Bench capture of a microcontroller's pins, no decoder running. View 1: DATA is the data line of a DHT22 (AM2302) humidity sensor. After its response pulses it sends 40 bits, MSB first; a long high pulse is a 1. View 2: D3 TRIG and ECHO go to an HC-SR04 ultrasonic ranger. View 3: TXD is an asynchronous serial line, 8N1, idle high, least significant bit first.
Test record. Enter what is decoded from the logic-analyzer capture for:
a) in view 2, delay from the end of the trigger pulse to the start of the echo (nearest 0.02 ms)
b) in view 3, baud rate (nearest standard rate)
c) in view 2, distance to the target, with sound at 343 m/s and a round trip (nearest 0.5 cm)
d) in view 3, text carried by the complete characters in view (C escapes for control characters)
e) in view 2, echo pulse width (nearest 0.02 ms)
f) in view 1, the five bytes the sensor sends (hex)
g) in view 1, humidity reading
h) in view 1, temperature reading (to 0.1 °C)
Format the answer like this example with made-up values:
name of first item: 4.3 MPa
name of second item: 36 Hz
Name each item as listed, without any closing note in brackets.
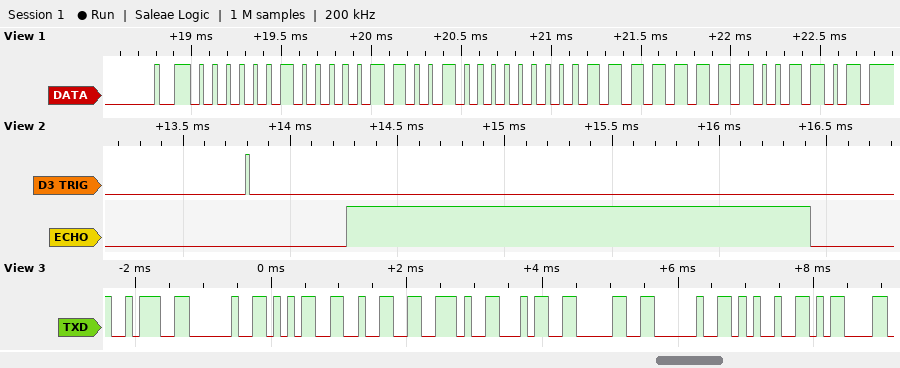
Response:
in view 2, delay from the end of the trigger pulse to the start of the echo: 0.46 ms
in view 3, baud rate: 9600 baud
in view 2, distance to the target, with sound at 343 m/s and a round trip: 37 cm
in view 3, text carried by the complete characters in view: ": 52.40 %\r"
in view 2, echo pulse width: 2.16 ms
in view 1, the five bytes the sensor sends: 02 0C 80 3F CD
in view 1, humidity reading: 52.4 %
in view 1, temperature reading: -6.3 °C
